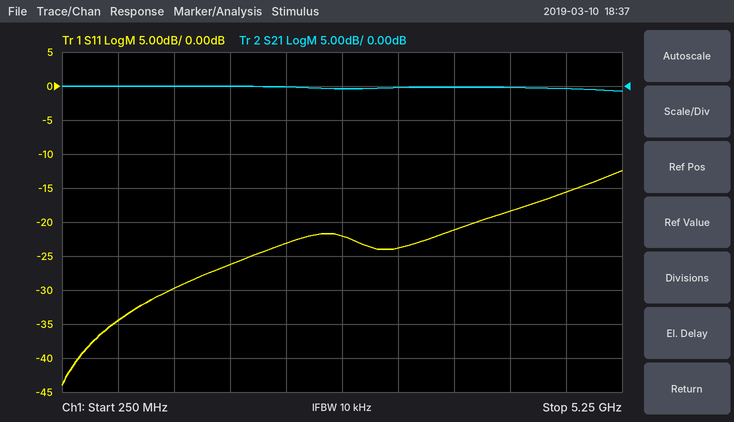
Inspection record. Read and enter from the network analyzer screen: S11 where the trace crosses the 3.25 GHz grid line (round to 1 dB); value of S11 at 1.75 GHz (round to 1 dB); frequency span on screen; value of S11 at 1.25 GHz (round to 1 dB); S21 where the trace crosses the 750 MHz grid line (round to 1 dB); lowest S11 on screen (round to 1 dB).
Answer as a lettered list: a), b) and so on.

a) -24 dB
b) -26 dB
c) 5 GHz
d) -30 dB
e) 0 dB
f) -44 dB
